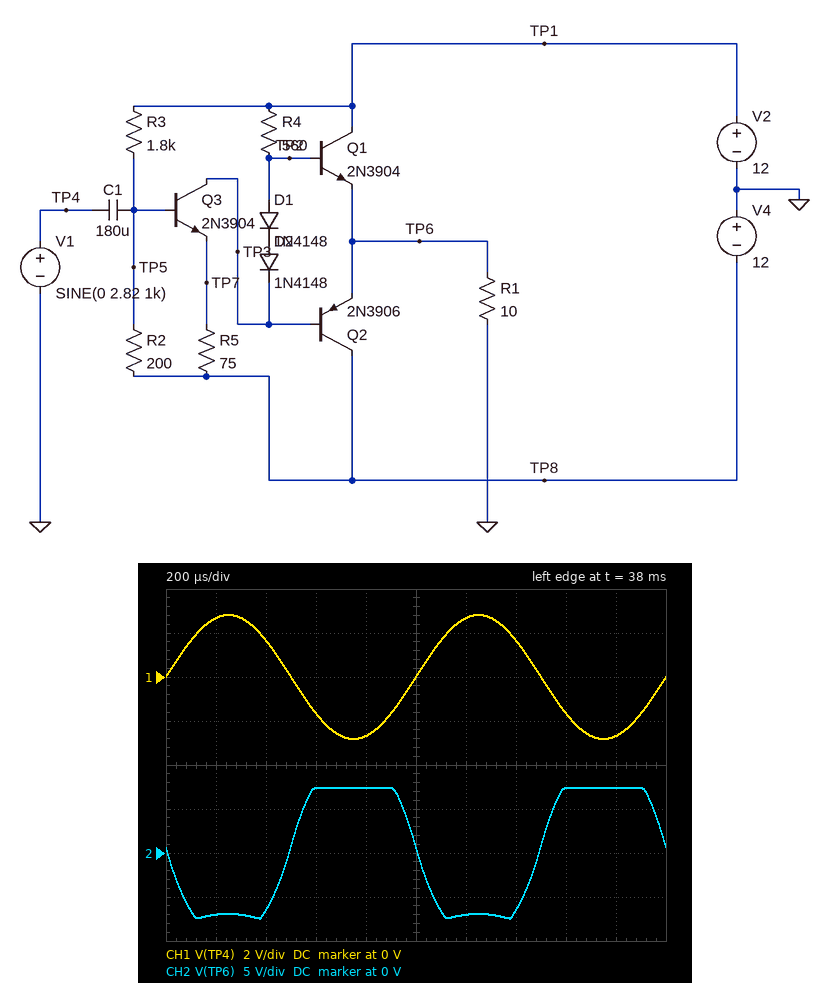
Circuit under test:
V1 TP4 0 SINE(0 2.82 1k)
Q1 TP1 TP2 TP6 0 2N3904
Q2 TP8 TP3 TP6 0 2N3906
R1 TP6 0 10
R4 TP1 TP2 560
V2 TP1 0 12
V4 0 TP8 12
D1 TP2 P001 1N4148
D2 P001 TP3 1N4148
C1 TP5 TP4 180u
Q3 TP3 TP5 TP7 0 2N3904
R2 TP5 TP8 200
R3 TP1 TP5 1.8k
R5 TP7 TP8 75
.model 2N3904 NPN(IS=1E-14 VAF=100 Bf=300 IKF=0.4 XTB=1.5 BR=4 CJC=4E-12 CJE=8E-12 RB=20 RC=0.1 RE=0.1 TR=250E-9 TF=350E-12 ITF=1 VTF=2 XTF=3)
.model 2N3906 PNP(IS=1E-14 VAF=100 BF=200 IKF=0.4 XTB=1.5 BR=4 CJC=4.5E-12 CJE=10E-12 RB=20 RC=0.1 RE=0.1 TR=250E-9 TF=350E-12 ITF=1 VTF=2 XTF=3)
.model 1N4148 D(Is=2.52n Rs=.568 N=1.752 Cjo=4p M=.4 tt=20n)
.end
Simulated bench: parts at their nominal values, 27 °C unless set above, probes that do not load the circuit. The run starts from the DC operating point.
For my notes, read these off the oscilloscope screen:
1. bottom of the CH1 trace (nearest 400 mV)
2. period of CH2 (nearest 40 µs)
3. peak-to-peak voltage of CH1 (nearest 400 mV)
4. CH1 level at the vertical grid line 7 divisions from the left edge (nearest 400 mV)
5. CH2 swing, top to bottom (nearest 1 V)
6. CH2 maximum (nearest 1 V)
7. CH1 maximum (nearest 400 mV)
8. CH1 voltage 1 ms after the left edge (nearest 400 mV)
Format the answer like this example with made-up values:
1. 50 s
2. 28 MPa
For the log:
1. -2.8 V
2. 1.00 ms
3. 5.6 V
4. 1.6 V
5. 15 V
6. 7 V
7. 2.8 V
8. 0 V
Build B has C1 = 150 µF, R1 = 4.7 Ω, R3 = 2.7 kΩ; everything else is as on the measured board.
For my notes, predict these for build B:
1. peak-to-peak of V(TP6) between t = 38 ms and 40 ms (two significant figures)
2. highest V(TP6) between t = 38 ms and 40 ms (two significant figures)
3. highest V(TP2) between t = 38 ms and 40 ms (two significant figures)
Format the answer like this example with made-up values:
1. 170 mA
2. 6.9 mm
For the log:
1. 10 V
2. 4.8 V
3. 6.0 V
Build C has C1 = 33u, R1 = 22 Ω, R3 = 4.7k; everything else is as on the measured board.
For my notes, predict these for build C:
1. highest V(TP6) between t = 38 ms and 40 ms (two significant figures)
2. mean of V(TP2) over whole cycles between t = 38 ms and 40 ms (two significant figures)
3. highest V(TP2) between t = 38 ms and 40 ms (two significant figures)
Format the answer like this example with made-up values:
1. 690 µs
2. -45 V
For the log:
1. 9.5 V
2. 4.1 V
3. 10 V
